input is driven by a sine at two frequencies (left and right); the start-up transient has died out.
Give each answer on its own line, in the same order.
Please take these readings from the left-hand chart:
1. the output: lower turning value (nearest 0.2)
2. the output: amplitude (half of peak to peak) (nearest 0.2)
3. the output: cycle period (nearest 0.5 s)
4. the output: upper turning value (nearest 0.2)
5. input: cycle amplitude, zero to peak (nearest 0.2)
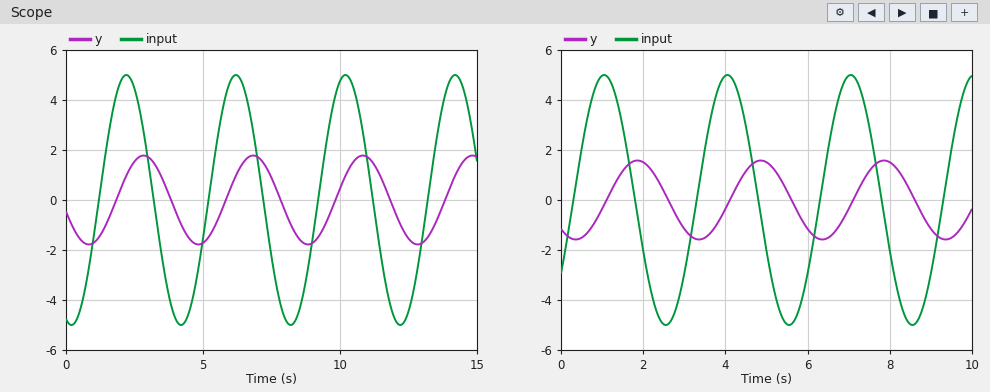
-1.8
1.8
4.0 s
1.8
5.0
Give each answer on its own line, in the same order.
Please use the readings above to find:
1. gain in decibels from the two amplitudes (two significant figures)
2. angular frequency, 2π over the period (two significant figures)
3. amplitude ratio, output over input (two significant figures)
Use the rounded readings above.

-8.9 dB
1.6 rad/s
0.36
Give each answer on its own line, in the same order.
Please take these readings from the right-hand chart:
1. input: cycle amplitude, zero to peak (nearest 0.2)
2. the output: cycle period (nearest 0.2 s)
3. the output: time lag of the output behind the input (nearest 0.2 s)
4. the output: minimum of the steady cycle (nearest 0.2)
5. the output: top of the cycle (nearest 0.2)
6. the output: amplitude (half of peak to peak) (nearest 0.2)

5.0
3.0 s
0.8 s
-1.6
1.6
1.6
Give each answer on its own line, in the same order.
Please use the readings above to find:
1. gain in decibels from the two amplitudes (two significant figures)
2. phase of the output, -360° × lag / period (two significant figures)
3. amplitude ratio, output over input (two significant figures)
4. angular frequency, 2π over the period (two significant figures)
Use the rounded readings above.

-9.9 dB
-96°
0.32
2.1 rad/s
